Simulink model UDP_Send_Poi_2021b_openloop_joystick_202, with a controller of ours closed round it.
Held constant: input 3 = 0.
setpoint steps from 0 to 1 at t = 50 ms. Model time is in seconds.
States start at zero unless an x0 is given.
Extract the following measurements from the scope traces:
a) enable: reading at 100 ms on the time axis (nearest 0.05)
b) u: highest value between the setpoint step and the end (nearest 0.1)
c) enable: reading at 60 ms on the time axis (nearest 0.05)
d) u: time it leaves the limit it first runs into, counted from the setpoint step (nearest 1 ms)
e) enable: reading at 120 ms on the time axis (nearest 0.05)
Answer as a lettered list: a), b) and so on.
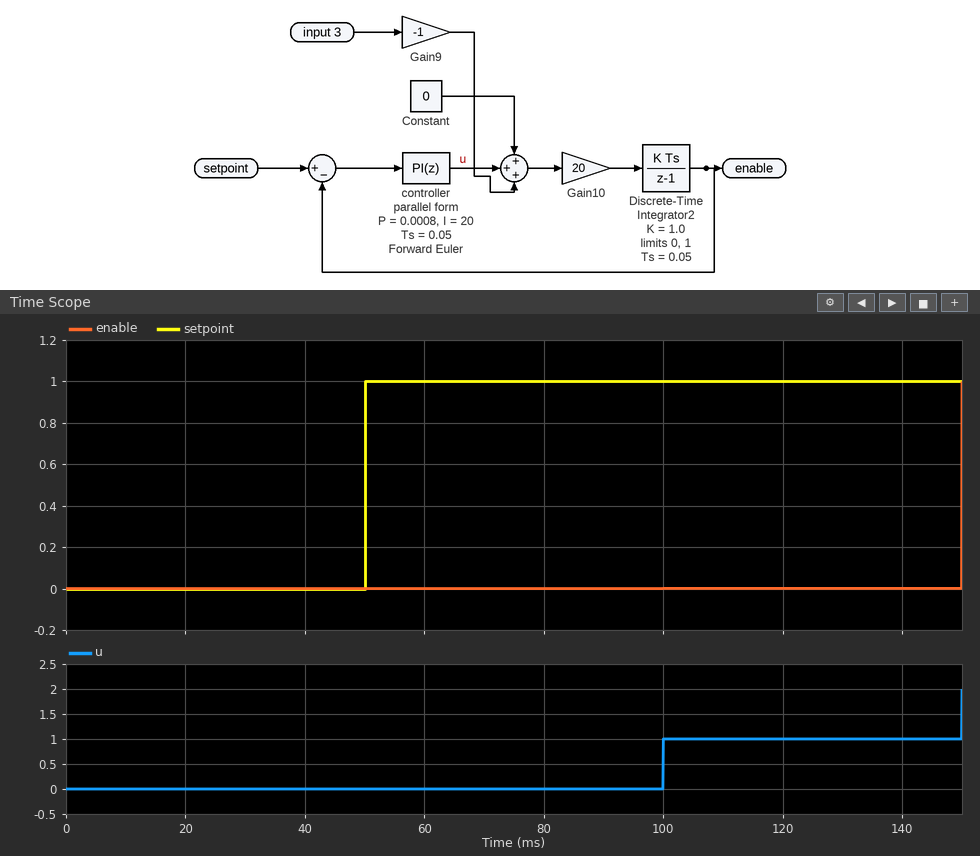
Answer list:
a) 0.00
b) 1.0
c) 0.00
d) 50 ms
e) 0.00
